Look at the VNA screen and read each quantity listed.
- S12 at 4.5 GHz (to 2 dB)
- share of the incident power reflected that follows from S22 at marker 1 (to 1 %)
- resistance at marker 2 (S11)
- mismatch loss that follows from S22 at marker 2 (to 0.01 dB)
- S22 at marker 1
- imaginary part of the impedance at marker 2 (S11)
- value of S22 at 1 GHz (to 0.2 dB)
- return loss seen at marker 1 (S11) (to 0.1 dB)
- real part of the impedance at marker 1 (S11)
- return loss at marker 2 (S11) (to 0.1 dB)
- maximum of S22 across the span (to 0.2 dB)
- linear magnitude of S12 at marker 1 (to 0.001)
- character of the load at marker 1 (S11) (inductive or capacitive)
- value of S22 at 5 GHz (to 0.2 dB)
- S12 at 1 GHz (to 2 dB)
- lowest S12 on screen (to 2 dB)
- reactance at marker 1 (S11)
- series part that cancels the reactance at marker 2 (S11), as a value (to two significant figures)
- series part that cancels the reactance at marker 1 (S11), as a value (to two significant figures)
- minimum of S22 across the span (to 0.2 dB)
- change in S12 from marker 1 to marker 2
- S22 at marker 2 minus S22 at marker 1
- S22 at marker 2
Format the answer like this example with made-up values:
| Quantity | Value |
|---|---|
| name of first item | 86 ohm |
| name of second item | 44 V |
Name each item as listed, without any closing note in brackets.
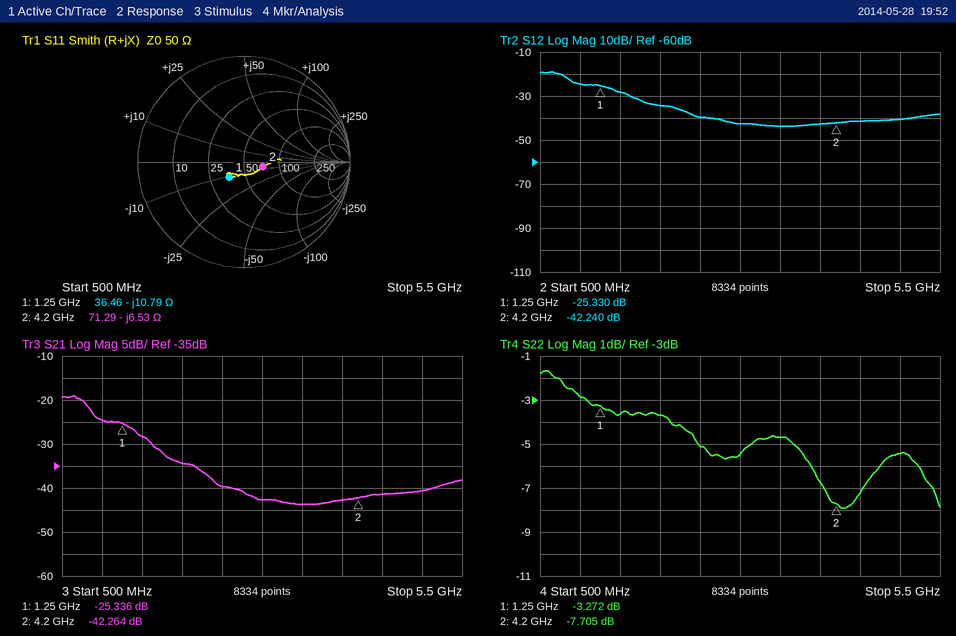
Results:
| Quantity | Value |
|---|---|
| S12 at 4.5 GHz | -42 dB |
| share of the incident power reflected that follows from S22 at marker 1 | 47 % |
| resistance at marker 2 | 71.29 Ω |
| mismatch loss that follows from S22 at marker 2 | 0.81 dB |
| S22 at marker 1 | -3.272 dB |
| imaginary part of the impedance at marker 2 | -6.53 Ω |
| value of S22 at 1 GHz | -2.8 dB |
| return loss seen at marker 1 (S11) | 14.0 dB |
| real part of the impedance at marker 1 | 36.46 Ω |
| return loss at marker 2 (S11) | 14.7 dB |
| maximum of S22 across the span | -1.6 dB |
| linear magnitude of S12 at marker 1 | 0.054 |
| character of the load at marker 1 (S11) | capacitive |
| value of S22 at 5 GHz | -5.4 dB |
| S12 at 1 GHz | -24 dB |
| lowest S12 on screen | -44 dB |
| reactance at marker 1 | -10.79 Ω |
| series part that cancels the reactance at marker 2 (S11), as a value | 250 pH |
| series part that cancels the reactance at marker 1 (S11), as a value | 1.4 nH |
| minimum of S22 across the span | -8.0 dB |
| change in S12 from marker 1 to marker 2 | -16.910 dB |
| S22 at marker 2 minus S22 at marker 1 | -4.433 dB |
| S22 at marker 2 | -7.705 dB |
